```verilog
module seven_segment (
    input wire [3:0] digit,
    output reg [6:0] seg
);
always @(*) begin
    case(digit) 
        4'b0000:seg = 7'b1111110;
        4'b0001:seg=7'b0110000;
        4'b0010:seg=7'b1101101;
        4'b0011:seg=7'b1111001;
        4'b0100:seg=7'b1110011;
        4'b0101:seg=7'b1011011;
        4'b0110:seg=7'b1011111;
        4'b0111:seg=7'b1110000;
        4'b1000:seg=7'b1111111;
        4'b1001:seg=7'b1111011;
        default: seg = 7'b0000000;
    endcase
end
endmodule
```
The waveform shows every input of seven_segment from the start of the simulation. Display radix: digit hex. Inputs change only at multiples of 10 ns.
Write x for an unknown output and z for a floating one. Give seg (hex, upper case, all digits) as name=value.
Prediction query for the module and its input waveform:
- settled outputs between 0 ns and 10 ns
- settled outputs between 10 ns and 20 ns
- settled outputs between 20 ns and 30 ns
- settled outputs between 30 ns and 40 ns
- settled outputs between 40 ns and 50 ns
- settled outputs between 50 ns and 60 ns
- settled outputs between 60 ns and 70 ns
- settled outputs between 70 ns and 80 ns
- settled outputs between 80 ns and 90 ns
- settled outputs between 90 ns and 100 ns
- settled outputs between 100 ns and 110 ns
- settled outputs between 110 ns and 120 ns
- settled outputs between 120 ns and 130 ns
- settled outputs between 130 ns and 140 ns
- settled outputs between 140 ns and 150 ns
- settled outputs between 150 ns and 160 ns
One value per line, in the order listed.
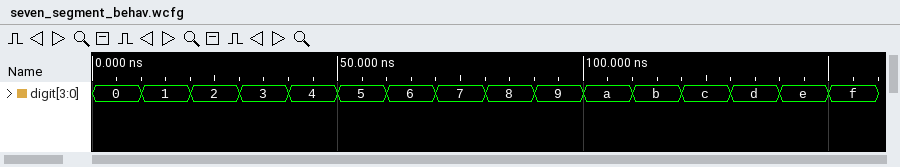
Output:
seg=7E
seg=30
seg=6D
seg=79
seg=73
seg=5B
seg=5F
seg=70
seg=7F
seg=7B
seg=00
seg=00
seg=00
seg=00
seg=00
seg=00
